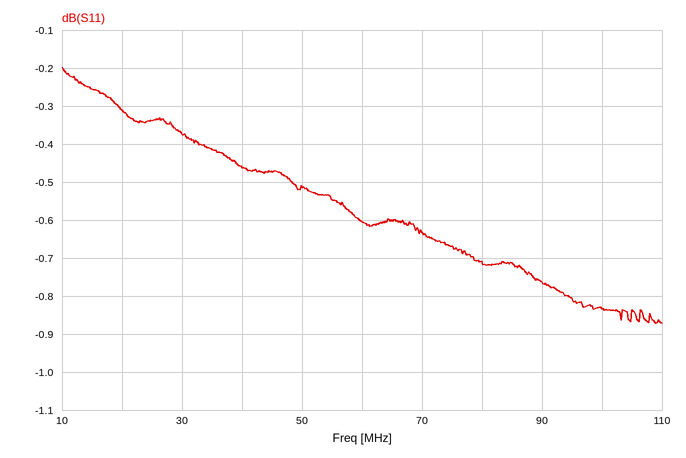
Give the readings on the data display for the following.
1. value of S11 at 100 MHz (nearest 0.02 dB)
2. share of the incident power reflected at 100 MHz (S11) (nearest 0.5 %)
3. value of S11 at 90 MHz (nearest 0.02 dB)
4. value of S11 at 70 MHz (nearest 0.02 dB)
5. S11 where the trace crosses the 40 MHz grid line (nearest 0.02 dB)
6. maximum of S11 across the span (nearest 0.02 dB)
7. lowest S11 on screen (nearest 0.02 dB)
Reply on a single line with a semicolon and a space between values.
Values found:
-0.84 dB; 82.5 %; -0.76 dB; -0.64 dB; -0.46 dB; -0.20 dB; -0.88 dB
